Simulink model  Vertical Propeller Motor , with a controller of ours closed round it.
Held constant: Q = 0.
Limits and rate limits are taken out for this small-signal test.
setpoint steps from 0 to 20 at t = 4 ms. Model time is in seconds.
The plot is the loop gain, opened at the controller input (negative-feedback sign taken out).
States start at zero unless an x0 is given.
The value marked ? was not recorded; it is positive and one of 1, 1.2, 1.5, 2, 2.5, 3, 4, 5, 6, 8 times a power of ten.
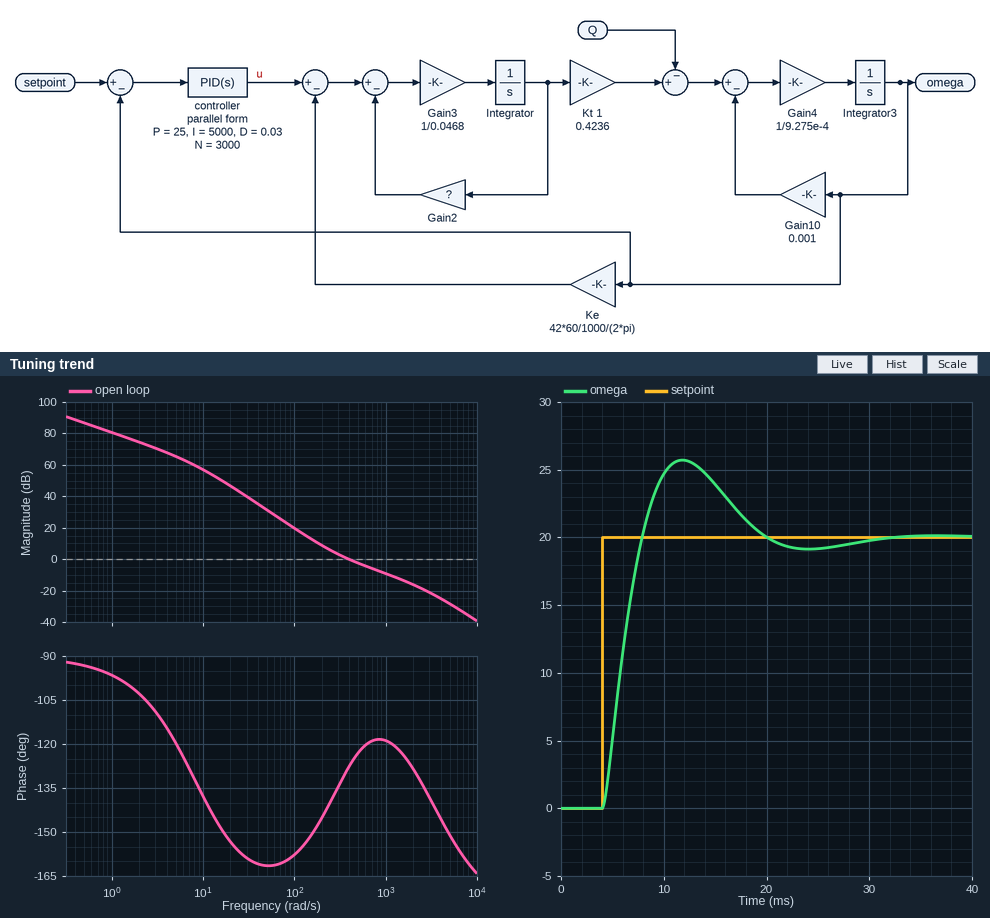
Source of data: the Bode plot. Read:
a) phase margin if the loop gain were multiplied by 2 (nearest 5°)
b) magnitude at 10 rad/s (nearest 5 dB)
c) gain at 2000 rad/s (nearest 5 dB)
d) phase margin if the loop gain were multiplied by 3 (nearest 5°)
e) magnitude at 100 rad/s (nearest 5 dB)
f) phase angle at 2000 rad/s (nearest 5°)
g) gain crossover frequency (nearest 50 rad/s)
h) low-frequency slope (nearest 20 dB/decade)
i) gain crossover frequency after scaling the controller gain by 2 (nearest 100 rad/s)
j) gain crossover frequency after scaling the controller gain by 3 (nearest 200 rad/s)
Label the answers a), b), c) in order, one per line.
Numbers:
a) 60°
b) 55 dB
c) -15 dB
d) 60°
e) 20 dB
f) -130°
g) 400 rad/s
h) -20 dB/decade
i) 700 rad/s
j) 1000 rad/s
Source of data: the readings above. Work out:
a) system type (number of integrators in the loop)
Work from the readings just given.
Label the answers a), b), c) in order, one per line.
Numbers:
a) 1
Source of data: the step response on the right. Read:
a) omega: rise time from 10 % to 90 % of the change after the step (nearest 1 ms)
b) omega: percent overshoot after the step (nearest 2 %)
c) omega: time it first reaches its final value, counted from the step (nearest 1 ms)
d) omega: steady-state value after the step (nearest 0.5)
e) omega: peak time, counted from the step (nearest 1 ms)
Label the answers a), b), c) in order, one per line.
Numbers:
a) 3 ms
b) 28 %
c) 4 ms
d) 20.0
e) 8 ms
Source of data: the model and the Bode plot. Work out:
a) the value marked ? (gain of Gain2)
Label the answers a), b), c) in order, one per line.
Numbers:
a) 25
